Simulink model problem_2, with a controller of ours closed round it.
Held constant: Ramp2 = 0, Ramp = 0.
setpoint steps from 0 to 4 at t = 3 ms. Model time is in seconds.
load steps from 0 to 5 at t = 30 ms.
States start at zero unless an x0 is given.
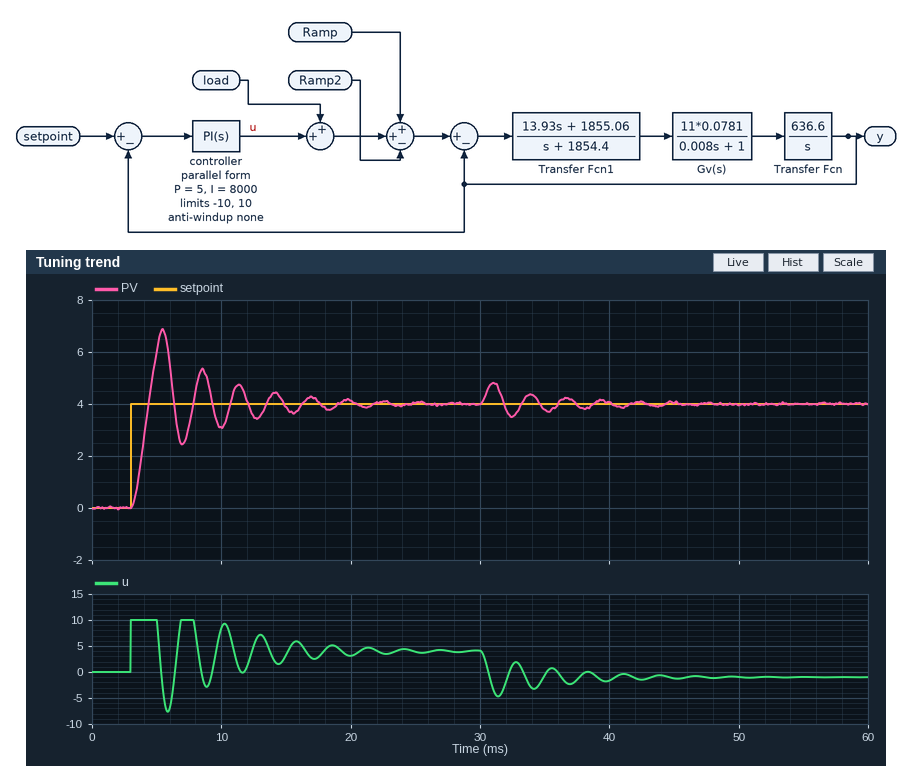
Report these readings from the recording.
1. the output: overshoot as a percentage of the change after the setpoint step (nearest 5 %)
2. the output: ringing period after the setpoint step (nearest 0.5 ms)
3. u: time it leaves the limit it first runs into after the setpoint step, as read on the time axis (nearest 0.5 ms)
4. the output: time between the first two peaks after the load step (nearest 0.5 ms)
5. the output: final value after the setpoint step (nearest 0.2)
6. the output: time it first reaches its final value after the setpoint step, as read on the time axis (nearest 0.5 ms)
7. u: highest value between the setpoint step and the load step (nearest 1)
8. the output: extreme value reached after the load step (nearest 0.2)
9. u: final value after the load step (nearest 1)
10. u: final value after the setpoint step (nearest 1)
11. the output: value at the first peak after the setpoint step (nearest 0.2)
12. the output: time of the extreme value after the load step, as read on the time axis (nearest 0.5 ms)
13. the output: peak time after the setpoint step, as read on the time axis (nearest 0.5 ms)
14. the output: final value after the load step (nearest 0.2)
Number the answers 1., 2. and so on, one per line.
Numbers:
1. 70 %
2. 3.0 ms
3. 5.0 ms
4. 3.0 ms
5. 4.0
6. 4.5 ms
7. 10
8. 4.8
9. -1
10. 4
11. 6.8
12. 31.0 ms
13. 5.5 ms
14. 4.0
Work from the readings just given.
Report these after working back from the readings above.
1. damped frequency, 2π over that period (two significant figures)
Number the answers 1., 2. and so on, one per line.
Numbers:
1. 2.1 rad/ms
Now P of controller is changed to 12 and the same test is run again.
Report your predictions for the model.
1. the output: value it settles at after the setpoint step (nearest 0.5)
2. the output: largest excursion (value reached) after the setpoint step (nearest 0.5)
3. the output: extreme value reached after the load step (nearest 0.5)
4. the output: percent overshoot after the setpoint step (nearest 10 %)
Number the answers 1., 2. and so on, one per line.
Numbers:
1. 4.0
2. 6.0
3. 4.5
4. 50 %
